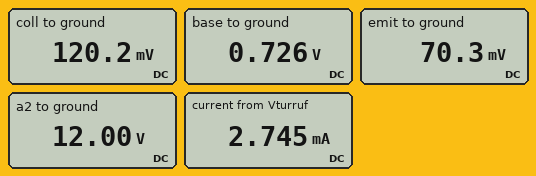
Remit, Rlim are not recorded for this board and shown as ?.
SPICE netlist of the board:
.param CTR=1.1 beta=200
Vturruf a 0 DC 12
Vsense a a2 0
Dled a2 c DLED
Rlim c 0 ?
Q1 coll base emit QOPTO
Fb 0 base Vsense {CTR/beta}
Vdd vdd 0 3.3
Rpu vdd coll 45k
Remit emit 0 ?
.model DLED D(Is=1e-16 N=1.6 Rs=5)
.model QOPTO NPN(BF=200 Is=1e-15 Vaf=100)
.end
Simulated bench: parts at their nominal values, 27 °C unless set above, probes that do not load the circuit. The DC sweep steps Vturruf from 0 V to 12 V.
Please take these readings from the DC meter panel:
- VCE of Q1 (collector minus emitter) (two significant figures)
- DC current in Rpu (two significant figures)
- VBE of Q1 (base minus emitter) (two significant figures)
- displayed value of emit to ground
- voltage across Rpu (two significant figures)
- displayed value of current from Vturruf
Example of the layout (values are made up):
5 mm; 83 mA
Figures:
50 mV; 71 µA; 660 mV; 70.3 mV; 3.2 V; 2.745 mA
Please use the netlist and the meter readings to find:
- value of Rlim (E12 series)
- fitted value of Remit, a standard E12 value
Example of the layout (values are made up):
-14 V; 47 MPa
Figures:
3.9 kΩ; 820 Ω
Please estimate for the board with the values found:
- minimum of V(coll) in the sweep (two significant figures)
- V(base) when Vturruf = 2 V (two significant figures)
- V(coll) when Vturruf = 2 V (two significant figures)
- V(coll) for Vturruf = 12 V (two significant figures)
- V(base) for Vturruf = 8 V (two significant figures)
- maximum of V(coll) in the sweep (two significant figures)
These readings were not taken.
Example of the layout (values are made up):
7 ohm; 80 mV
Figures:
120 mV; 700 mV; 170 mV; 120 mV; 720 mV; 3.3 V
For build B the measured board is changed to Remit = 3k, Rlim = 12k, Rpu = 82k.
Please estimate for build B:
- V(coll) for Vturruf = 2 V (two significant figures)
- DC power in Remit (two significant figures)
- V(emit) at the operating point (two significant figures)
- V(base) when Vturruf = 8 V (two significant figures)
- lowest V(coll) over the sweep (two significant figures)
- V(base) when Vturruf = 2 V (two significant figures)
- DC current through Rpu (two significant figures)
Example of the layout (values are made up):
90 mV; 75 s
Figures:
250 mV; 5.5 µW; 130 mV; 760 mV; 190 mV; 740 mV; 38 µA
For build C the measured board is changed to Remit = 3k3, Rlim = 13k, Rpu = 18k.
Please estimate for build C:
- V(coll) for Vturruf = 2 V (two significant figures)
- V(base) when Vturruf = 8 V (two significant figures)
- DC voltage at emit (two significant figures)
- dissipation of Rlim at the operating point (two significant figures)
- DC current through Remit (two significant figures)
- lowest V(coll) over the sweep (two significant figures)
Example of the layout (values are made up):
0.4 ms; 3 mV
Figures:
2.0 V; 1.2 V; 510 mV; 8.9 mW; 150 µA; 610 mV
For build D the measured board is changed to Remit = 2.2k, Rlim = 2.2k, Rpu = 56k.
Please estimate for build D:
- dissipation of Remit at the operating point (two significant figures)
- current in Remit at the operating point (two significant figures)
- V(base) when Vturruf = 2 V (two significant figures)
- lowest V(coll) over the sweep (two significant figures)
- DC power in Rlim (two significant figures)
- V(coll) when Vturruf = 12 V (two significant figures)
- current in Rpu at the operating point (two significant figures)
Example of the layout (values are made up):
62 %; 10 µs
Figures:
15 µW; 82 µA; 770 mV; 200 mV; 52 mW; 220 mV; 55 µA
